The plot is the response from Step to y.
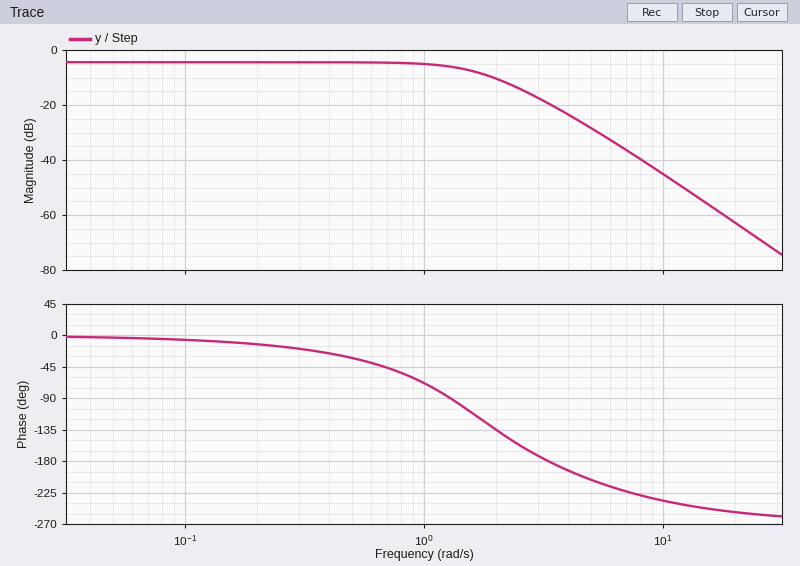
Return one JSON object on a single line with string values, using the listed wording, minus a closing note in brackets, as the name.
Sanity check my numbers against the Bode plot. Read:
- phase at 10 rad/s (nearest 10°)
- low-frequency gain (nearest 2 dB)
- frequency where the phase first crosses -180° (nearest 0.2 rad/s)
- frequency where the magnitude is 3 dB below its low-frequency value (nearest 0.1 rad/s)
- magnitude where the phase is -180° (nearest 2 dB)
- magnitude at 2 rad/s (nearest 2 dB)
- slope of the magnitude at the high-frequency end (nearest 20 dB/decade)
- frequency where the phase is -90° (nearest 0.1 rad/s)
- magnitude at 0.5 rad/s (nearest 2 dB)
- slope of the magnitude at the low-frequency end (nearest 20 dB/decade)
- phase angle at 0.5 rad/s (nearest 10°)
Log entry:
{"phase at 10 rad/s": "-240°", "low-frequency gain": "-4 dB", "frequency where the phase first crosses -180°": "3.4 rad/s", "frequency where the magnitude is 3 dB below its low-frequency value": "1.6 rad/s", "magnitude where the phase is -180°": "-20 dB", "magnitude at 2 rad/s": "-10 dB", "slope of the magnitude at the high-frequency end": "-60 dB/decade", "frequency where the phase is -90°": "1.3 rad/s", "magnitude at 0.5 rad/s": "-4 dB", "slope of the magnitude at the low-frequency end": "0 dB/decade", "phase angle at 0.5 rad/s": "-30°"}
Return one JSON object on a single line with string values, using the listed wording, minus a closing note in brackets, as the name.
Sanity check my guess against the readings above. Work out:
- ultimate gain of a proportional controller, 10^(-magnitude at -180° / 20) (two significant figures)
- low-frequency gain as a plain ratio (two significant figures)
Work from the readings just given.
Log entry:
{"ultimate gain of a proportional controller, 10^(-magnitude at -180° / 20)": "10", "low-frequency gain as a plain ratio": "0.63"}
